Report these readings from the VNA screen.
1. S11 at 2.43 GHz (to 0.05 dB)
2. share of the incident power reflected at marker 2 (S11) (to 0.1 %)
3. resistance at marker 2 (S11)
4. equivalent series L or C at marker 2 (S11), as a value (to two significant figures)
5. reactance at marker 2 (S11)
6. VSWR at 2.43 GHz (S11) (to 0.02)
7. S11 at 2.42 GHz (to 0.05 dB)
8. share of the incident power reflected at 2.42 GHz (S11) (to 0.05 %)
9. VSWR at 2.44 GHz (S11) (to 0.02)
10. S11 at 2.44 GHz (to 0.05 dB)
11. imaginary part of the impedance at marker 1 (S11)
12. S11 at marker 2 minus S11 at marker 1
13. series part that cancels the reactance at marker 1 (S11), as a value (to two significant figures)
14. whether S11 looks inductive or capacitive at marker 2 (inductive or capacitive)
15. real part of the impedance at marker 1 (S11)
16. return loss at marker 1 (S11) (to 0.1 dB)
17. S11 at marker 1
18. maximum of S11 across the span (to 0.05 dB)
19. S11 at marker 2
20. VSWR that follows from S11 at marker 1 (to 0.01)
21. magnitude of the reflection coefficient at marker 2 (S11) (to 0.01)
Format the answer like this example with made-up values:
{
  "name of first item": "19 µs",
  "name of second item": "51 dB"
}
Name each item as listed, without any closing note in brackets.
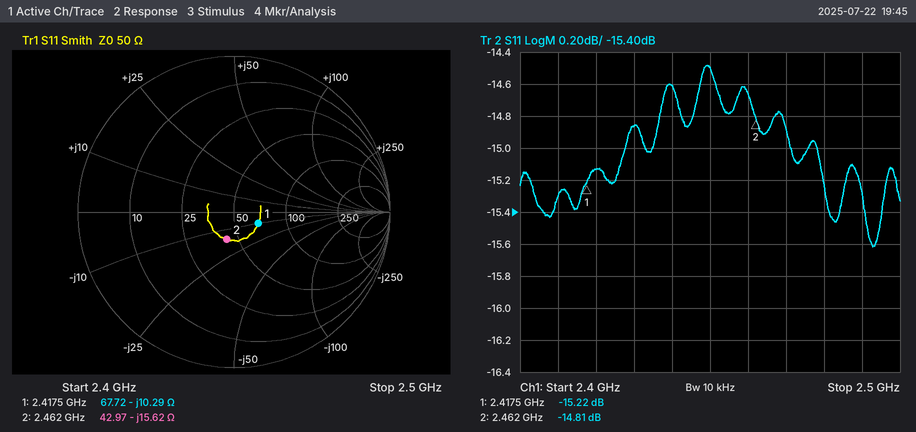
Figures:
{
  "S11 at 2.43 GHz": "-14.85 dB",
  "share of the incident power reflected at marker 2 (S11)": "3.3 %",
  "resistance at marker 2": "42.97 Ω",
  "equivalent series L or C at marker 2 (S11), as a value": "4.1 pF",
  "reactance at marker 2": "-15.62 Ω",
  "VSWR at 2.43 GHz (S11)": "1.44",
  "S11 at 2.42 GHz": "-15.15 dB",
  "share of the incident power reflected at 2.42 GHz (S11)": "3.05 %",
  "VSWR at 2.44 GHz (S11)": "1.46",
  "S11 at 2.44 GHz": "-14.60 dB",
  "imaginary part of the impedance at marker 1": "-10.29 Ω",
  "S11 at marker 2 minus S11 at marker 1": "0.41 dB",
  "series part that cancels the reactance at marker 1 (S11), as a value": "680 pH",
  "whether S11 looks inductive or capacitive at marker 2": "capacitive",
  "real part of the impedance at marker 1": "67.72 Ω",
  "return loss at marker 1 (S11)": "15.2 dB",
  "S11 at marker 1": "-15.22 dB",
  "maximum of S11 across the span": "-14.50 dB",
  "S11 at marker 2": "-14.81 dB",
  "VSWR that follows from S11 at marker 1": "1.42",
  "magnitude of the reflection coefficient at marker 2 (S11)": "0.18"
}
